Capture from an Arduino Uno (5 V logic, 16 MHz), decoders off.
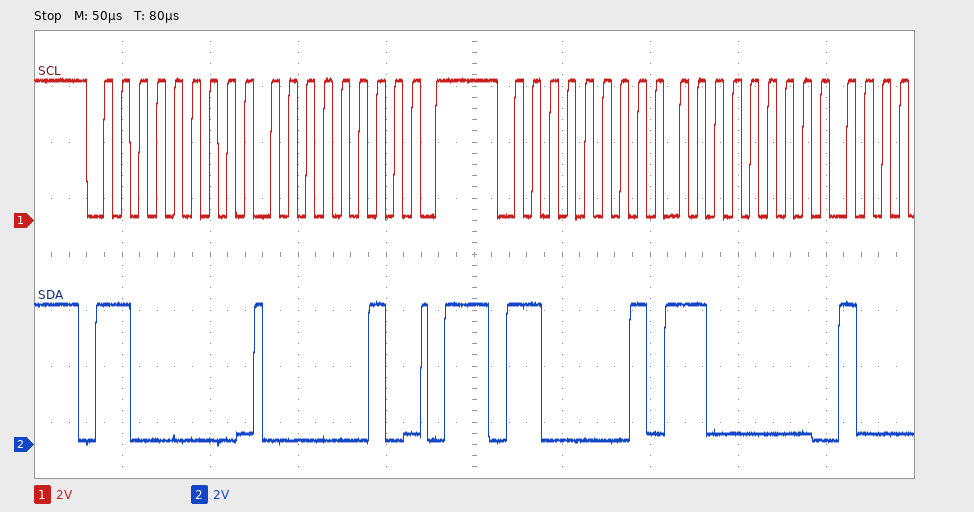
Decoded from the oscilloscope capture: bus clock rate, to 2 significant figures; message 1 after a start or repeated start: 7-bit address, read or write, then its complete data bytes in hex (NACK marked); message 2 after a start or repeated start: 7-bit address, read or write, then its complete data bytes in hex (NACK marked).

100 kHz
0x60 write: 02
0x60 read: C0
